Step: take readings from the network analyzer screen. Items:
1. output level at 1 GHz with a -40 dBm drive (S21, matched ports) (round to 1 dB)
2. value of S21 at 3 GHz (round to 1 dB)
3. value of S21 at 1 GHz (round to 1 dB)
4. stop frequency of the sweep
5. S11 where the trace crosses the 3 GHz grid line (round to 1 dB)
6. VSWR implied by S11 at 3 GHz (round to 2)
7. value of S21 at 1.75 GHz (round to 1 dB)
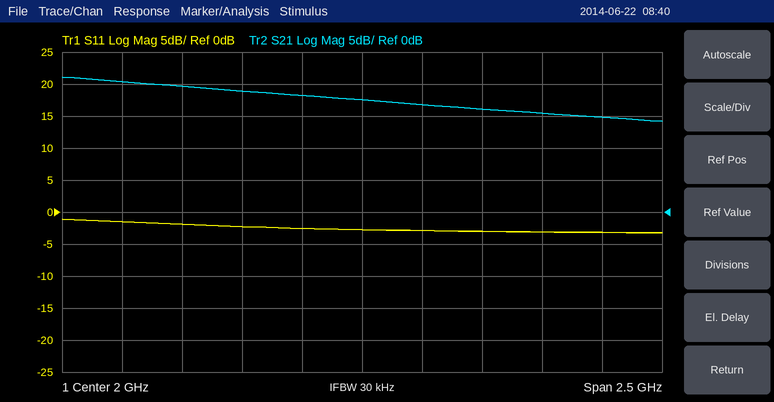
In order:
-20 dBm
15 dB
20 dB
3.25 GHz
-3 dB
6
18 dB
